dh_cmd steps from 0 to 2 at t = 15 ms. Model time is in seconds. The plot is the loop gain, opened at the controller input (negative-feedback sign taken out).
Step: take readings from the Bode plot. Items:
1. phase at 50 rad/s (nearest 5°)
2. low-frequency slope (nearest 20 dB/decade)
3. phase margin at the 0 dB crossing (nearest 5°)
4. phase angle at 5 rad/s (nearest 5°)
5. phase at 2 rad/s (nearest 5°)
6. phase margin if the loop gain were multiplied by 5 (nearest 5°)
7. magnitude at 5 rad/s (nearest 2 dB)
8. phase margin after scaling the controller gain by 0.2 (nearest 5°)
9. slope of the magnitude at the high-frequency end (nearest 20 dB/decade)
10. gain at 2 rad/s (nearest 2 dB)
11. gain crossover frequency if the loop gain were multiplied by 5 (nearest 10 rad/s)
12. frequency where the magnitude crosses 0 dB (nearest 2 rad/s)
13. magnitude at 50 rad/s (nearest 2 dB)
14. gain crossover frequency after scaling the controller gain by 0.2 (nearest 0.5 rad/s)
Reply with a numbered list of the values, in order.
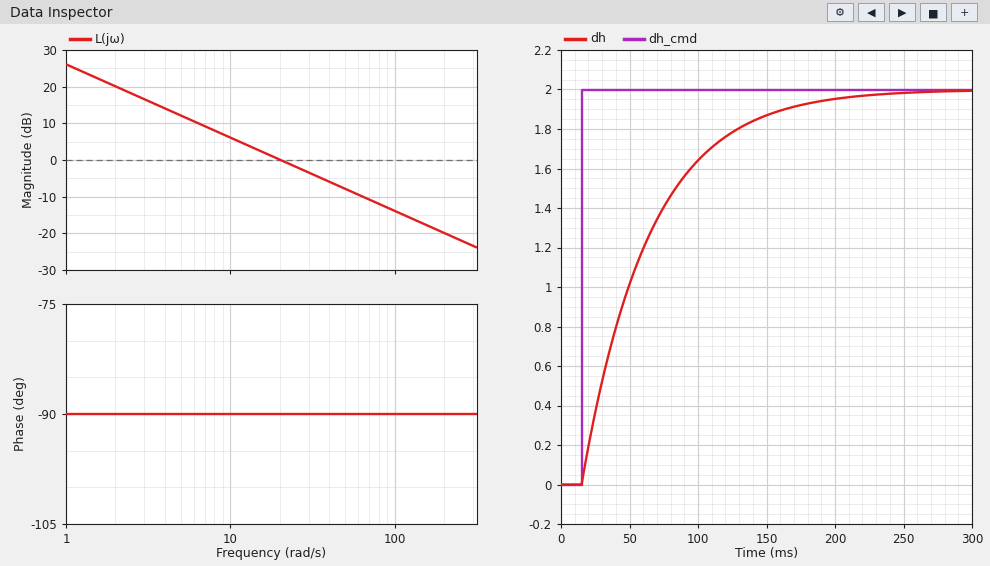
1. -90°
2. -20 dB/decade
3. 90°
4. -90°
5. -90°
6. 90°
7. 12 dB
8. 90°
9. -20 dB/decade
10. 20 dB
11. 100 rad/s
12. 20 rad/s
13. -8 dB
14. 4.0 rad/s
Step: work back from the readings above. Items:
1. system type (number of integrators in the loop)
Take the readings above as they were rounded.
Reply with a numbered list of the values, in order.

1. 1
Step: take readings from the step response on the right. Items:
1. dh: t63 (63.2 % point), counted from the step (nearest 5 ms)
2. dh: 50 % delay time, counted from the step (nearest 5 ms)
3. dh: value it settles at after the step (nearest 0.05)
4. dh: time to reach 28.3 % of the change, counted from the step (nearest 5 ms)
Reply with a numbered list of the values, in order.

1. 50 ms
2. 35 ms
3. 2.00
4. 15 ms
